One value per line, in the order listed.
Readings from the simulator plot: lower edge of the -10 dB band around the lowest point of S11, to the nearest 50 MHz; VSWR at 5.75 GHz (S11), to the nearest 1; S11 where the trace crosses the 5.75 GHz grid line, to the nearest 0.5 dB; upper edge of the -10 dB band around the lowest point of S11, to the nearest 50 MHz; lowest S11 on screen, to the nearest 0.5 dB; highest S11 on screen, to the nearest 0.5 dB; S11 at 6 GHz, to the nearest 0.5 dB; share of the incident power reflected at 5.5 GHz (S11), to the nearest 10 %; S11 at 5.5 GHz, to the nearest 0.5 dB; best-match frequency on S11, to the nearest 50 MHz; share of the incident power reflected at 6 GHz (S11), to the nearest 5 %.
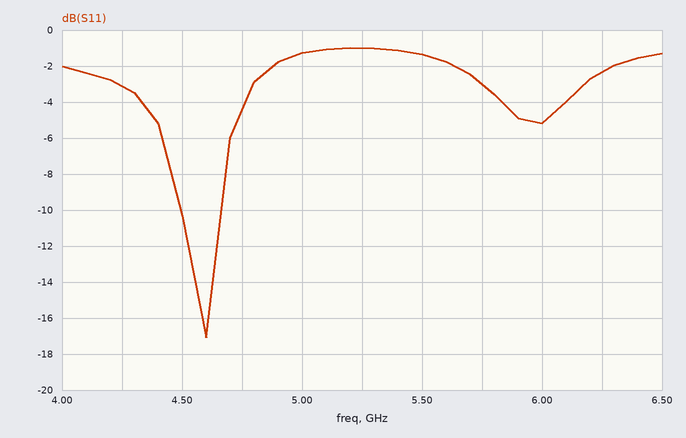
4.50 GHz
6
-3.0 dB
4.65 GHz
-17.0 dB
-1.0 dB
-5.0 dB
70 %
-1.5 dB
4.60 GHz
30 %
